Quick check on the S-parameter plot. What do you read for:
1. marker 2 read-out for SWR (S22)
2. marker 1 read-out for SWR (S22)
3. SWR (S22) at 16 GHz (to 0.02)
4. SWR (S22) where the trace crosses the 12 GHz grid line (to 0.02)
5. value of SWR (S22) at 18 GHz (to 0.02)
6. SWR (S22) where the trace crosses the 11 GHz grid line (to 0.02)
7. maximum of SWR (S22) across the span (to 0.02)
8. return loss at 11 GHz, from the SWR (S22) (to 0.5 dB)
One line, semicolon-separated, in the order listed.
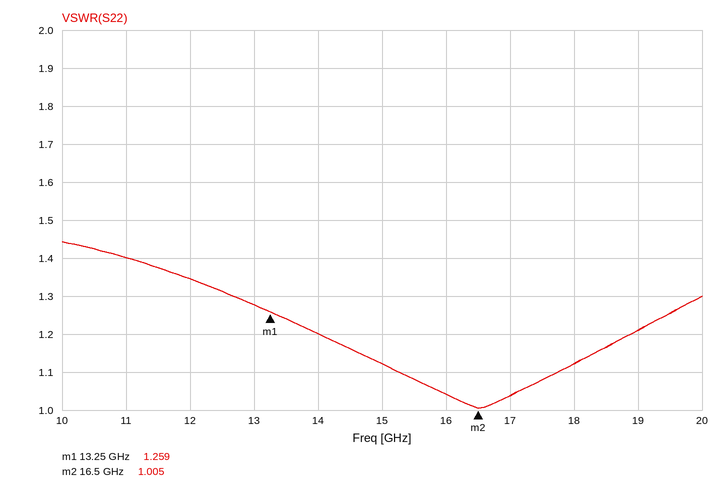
1.005; 1.259; 1.04; 1.34; 1.12; 1.40; 1.44; 15.5 dB
